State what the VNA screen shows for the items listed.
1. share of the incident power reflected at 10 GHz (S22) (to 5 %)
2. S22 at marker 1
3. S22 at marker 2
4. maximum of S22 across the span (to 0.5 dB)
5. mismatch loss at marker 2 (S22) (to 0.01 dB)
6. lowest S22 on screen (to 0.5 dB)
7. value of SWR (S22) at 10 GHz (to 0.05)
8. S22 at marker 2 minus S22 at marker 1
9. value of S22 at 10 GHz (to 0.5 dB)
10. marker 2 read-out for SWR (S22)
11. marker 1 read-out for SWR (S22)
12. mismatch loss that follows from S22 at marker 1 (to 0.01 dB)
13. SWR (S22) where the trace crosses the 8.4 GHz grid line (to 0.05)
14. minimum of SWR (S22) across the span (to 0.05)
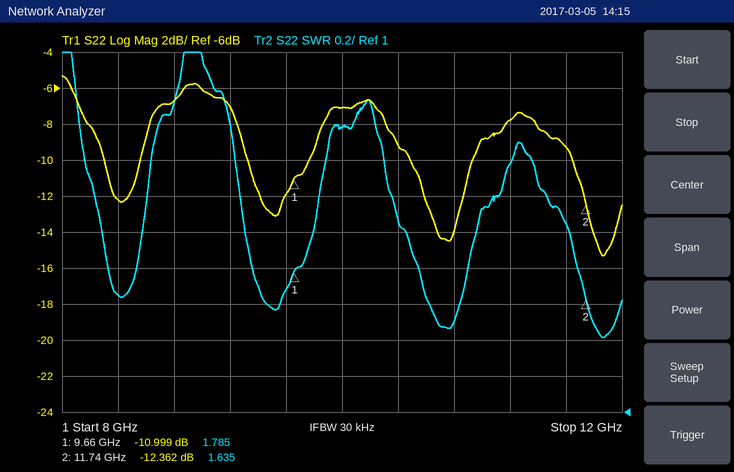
20 %
-10.999 dB
-12.362 dB
-5.5 dB
0.26 dB
-15.5 dB
2.60
-1.363 dB
-7.0 dB
1.635
1.785
0.36 dB
1.65
1.40
